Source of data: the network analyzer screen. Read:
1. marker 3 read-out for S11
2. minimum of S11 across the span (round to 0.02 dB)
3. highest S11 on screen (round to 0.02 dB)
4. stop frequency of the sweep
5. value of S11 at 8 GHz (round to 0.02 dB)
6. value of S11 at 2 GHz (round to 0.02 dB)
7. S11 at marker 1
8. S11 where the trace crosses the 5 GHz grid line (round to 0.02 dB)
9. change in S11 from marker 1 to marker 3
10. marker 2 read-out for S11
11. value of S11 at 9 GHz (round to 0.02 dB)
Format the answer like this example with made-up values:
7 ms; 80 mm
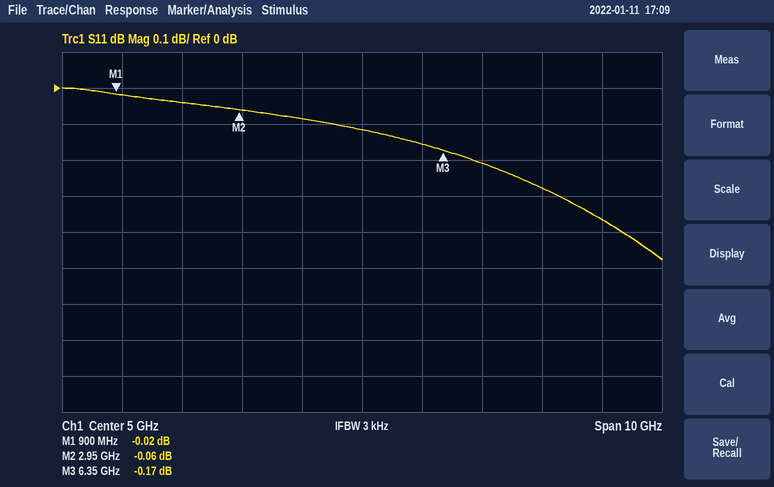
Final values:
-0.17 dB; -0.48 dB; 0.00 dB; 10 GHz; -0.28 dB; -0.04 dB; -0.02 dB; -0.12 dB; -0.15 dB; -0.06 dB; -0.36 dB
